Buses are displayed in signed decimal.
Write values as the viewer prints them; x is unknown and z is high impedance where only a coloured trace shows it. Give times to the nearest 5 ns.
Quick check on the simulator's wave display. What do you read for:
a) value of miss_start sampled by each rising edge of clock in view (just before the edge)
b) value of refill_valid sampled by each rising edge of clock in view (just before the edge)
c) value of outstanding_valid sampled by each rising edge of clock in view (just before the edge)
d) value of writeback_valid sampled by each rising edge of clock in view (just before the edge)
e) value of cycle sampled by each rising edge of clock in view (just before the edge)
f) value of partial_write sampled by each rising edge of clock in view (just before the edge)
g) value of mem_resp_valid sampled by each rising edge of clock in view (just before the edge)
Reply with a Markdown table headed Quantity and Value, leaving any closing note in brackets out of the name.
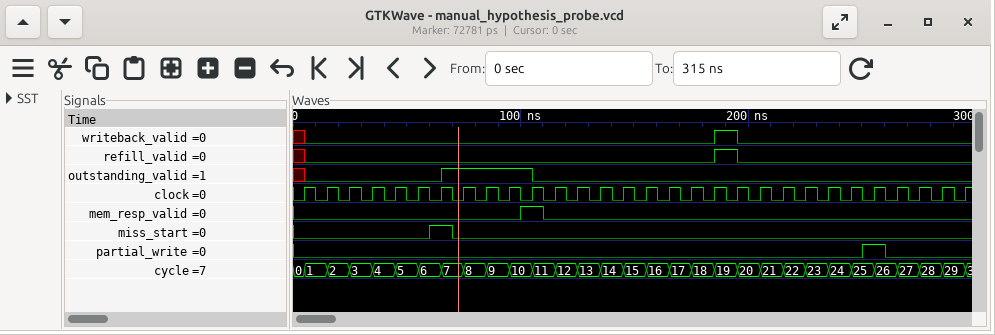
| Quantity | Value |
|---|---|
| value of miss_start sampled by each rising edge of clock in view | 0 0 0 0 0 0 1 0 0 0 0 0 0 0 0 0 0 0 0 0 0 0 0 0 0 0 0 0 0 0 |
| value of refill_valid sampled by each rising edge of clock in view | x 0 0 0 0 0 0 0 0 0 0 0 0 0 0 0 0 0 0 1 0 0 0 0 0 0 0 0 0 0 |
| value of outstanding_valid sampled by each rising edge of clock in view | x 0 0 0 0 0 0 1 1 1 1 0 0 0 0 0 0 0 0 0 0 0 0 0 0 0 0 0 0 0 |
| value of writeback_valid sampled by each rising edge of clock in view | x 0 0 0 0 0 0 0 0 0 0 0 0 0 0 0 0 0 0 1 0 0 0 0 0 0 0 0 0 0 |
| value of cycle sampled by each rising edge of clock in view | 0, 1, 2, 3, 4, 5, 6, 7, 8, 9, 10, 11, 12, 13, 14, 15, 16, 17, 18, 19, 20, 21, 22, 23, 24, 25, 26, 27, 28, 29 |
| value of partial_write sampled by each rising edge of clock in view | 0 0 0 0 0 0 0 0 0 0 0 0 0 0 0 0 0 0 0 0 0 0 0 0 0 1 0 0 0 0 |
| value of mem_resp_valid sampled by each rising edge of clock in view | 0 0 0 0 0 0 0 0 0 0 1 0 0 0 0 0 0 0 0 0 0 0 0 0 0 0 0 0 0 0 |
